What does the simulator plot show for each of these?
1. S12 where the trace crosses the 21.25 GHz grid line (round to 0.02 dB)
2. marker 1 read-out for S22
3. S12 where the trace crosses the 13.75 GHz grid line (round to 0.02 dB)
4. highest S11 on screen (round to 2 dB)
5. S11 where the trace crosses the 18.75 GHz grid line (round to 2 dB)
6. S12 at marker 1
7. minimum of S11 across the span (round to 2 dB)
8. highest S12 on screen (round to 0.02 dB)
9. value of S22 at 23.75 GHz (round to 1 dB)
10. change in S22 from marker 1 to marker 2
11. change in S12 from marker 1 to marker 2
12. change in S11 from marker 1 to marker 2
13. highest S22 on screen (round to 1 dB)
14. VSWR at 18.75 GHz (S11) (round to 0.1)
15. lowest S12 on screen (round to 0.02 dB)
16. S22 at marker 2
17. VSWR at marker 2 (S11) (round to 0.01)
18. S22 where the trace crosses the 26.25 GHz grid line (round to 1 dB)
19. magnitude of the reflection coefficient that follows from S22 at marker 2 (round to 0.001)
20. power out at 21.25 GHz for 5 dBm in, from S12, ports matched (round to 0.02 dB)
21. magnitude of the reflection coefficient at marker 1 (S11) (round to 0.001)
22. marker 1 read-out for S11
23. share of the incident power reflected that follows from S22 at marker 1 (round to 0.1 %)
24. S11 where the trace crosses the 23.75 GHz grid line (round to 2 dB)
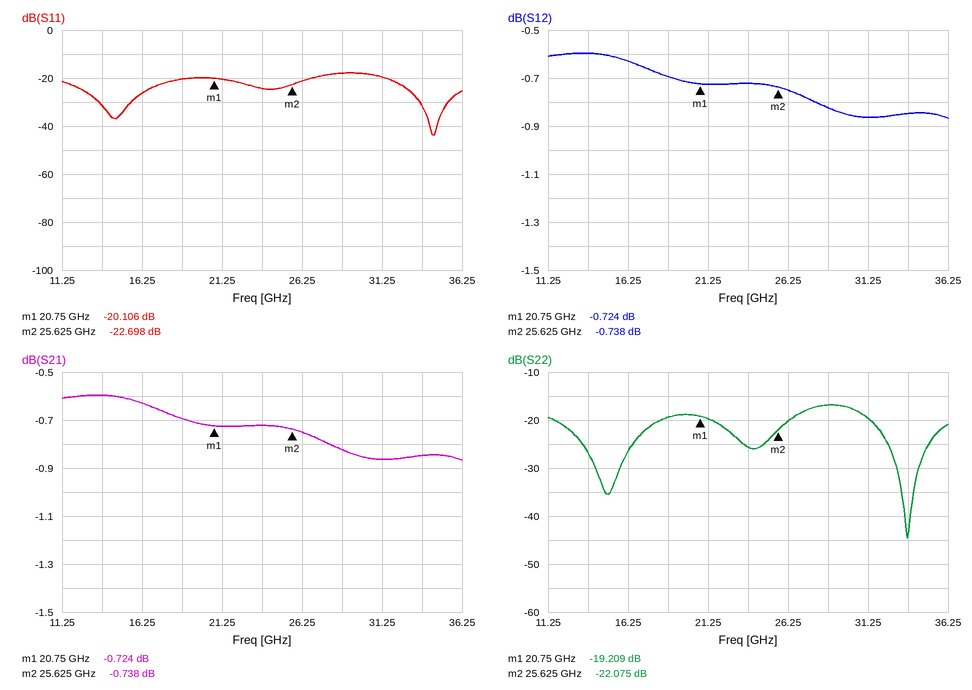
-0.72 dB
-19.209 dB
-0.60 dB
-18 dB
-20 dB
-0.724 dB
-44 dB
-0.60 dB
-26 dB
-2.866 dB
-0.014 dB
-2.592 dB
-17 dB
1.2
-0.86 dB
-22.075 dB
1.16
-20 dB
0.079
4.28 dBm
0.099
-20.106 dB
1.2 %
-24 dB
